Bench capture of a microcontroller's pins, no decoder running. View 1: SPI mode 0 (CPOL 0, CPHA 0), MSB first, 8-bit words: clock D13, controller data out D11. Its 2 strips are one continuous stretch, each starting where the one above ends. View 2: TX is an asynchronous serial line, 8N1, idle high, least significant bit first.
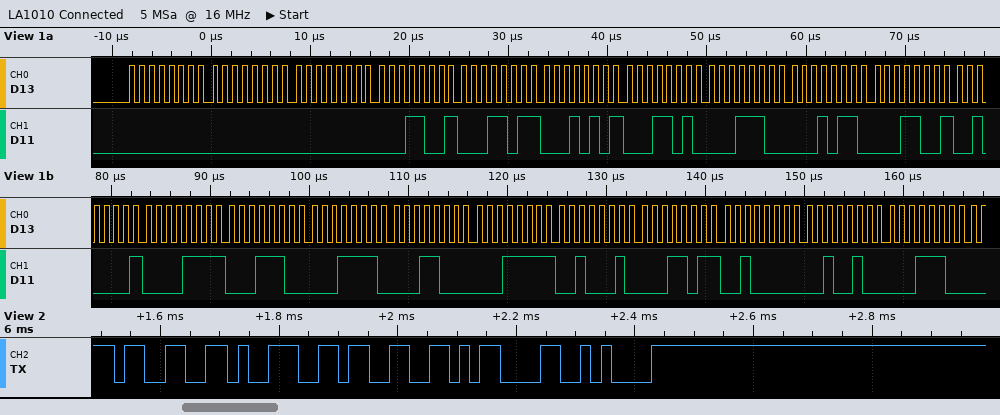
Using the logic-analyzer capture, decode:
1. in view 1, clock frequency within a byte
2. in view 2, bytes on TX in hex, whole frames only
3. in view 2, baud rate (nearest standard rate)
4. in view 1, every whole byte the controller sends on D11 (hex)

1 MHz
33 39 33 0D 0A
57600 baud
00 00 00 19 1B 15 1A 1C 16 19 21 0F 1C 1E 18 1F 22 1B 20 24 1C
